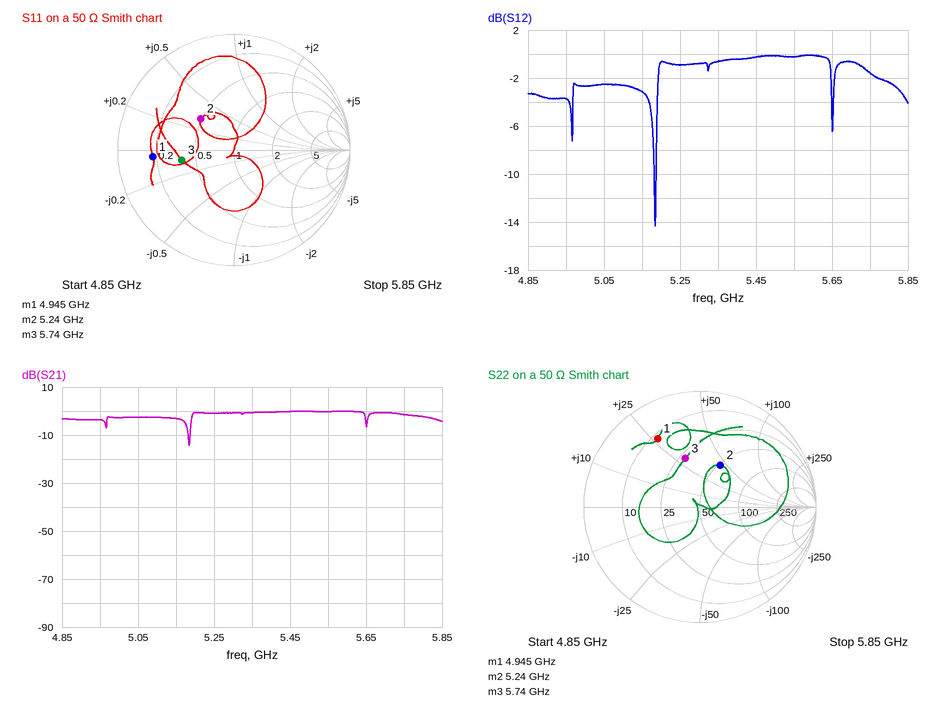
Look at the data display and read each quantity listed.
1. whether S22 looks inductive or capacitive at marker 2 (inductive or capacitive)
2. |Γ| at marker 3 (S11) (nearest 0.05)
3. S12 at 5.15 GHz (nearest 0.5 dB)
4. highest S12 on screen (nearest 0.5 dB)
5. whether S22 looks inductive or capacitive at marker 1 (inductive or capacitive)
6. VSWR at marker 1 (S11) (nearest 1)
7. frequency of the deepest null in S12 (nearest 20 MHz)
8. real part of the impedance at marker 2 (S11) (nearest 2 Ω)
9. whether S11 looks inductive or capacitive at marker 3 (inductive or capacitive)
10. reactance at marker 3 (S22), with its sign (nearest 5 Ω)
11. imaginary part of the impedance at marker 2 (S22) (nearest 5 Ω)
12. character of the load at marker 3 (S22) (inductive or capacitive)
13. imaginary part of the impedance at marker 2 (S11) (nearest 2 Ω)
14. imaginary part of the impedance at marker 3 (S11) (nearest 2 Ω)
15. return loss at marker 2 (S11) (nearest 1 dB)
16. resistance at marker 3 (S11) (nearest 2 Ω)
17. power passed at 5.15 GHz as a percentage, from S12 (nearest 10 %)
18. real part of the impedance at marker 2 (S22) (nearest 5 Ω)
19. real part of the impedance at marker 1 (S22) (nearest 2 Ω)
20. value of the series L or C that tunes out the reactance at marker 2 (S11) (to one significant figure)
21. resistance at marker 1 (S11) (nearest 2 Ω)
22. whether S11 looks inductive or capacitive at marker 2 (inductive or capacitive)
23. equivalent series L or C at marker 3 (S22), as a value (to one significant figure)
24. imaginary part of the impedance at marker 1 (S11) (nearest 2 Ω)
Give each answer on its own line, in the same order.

inductive
0.45
-3.0 dB
0.0 dB
inductive
6
5.18 GHz
24 Ω
capacitive
+30 Ω
+45 Ω
inductive
+16 Ω
-4 Ω
8 dB
18 Ω
50 %
50 Ω
12 Ω
2 pF
8 Ω
inductive
800 pH
-2 Ω
